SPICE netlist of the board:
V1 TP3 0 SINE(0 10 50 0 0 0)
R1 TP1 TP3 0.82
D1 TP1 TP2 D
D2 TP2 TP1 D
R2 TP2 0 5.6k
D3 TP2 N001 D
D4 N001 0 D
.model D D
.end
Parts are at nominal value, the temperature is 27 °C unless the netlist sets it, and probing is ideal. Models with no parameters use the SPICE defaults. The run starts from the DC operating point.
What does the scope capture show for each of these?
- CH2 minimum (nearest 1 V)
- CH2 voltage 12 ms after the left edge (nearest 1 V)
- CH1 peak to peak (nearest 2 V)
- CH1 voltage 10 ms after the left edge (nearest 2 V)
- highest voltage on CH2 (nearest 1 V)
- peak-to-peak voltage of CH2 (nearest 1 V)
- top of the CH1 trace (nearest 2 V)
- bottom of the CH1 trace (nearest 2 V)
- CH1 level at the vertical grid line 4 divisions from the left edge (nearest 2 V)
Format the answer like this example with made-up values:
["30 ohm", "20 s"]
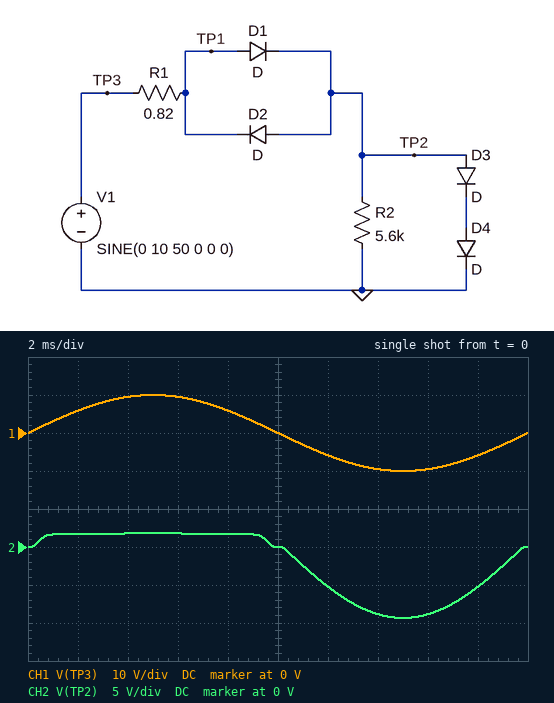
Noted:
["-9 V", "-5 V", "20 V", "0 V", "2 V", "11 V", "10 V", "-10 V", "6 V"]
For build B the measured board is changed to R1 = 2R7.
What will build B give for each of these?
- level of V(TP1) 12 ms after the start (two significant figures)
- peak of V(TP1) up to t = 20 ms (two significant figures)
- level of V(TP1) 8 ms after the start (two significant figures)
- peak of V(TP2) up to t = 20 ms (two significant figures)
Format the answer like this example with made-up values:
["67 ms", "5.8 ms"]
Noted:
["-5.9 V", "2.6 V", "2.5 V", "1.7 V"]
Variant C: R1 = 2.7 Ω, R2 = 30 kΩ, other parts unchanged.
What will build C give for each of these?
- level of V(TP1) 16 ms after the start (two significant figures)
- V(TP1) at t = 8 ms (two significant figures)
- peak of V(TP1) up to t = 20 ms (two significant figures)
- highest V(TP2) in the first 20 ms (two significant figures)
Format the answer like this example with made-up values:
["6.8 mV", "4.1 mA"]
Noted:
["-9.5 V", "2.5 V", "2.6 V", "1.7 V"]
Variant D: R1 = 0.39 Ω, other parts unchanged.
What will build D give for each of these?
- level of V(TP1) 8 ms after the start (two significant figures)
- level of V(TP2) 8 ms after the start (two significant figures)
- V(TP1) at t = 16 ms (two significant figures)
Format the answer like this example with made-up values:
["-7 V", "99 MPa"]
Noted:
["2.7 V", "1.8 V", "-9.5 V"]
